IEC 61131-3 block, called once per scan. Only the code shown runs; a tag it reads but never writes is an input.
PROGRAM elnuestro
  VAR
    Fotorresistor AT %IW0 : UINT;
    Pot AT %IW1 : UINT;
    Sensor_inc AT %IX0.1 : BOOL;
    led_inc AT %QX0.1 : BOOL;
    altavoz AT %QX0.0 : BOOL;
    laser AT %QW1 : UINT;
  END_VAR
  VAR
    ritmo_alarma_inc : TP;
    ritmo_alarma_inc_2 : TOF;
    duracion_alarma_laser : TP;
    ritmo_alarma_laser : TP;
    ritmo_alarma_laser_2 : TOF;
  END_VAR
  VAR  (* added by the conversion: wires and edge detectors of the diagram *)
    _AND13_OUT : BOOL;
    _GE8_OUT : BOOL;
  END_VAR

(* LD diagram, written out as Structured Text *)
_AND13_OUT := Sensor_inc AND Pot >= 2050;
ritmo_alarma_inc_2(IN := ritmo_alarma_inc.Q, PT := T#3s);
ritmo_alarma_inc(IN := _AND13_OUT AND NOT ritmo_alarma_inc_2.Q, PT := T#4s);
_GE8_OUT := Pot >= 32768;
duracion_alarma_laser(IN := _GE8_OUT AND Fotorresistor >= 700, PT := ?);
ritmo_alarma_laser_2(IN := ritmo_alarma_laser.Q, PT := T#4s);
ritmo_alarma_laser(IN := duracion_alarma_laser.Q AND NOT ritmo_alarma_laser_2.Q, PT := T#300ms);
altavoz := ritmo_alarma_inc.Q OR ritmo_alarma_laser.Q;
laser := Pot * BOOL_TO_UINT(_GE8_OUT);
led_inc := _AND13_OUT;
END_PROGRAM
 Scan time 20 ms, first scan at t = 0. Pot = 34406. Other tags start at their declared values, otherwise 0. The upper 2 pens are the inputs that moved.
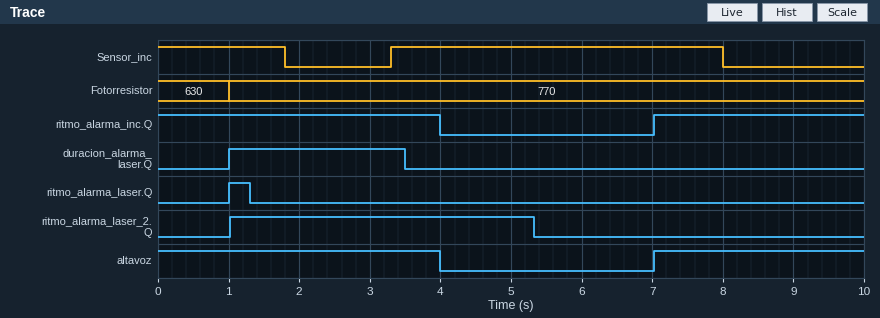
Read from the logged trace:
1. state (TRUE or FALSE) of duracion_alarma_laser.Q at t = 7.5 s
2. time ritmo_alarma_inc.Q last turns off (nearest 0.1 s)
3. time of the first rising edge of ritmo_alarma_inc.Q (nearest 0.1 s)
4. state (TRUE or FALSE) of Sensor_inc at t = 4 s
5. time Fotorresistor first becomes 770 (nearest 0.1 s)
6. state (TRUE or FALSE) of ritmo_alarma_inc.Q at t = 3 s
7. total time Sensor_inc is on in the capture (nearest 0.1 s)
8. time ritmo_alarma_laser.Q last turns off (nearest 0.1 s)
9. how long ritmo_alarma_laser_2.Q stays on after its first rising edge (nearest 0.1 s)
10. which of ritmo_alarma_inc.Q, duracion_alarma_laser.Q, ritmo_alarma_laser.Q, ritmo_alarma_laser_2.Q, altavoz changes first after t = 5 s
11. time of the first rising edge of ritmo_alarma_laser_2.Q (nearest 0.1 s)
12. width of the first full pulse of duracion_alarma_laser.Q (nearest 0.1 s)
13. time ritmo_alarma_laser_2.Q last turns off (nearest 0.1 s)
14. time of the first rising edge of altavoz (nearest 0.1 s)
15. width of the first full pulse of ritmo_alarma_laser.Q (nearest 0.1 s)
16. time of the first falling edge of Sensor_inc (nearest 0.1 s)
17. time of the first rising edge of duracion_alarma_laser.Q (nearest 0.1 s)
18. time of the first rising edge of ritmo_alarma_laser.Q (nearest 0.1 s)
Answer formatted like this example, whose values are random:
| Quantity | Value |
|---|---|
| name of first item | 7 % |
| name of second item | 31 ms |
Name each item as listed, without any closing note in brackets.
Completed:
| Quantity | Value |
|---|---|
| state (TRUE or FALSE) of duracion_alarma_laser.Q at t = 7.5 s | FALSE |
| time ritmo_alarma_inc.Q last turns off | 4.0 s |
| time of the first rising edge of ritmo_alarma_inc.Q | 7.0 s |
| state (TRUE or FALSE) of Sensor_inc at t = 4 s | TRUE |
| time Fotorresistor first becomes 770 | 1.0 s |
| state (TRUE or FALSE) of ritmo_alarma_inc.Q at t = 3 s | TRUE |
| total time Sensor_inc is on in the capture | 6.5 s |
| time ritmo_alarma_laser.Q last turns off | 1.3 s |
| how long ritmo_alarma_laser_2.Q stays on after its first rising edge | 4.3 s |
| which of ritmo_alarma_inc.Q, duracion_alarma_laser.Q, ritmo_alarma_laser.Q, ritmo_alarma_laser_2.Q, altavoz changes first after t = 5 s | ritmo_alarma_laser_2.Q |
| time of the first rising edge of ritmo_alarma_laser_2.Q | 1.0 s |
| width of the first full pulse of duracion_alarma_laser.Q | 2.5 s |
| time ritmo_alarma_laser_2.Q last turns off | 5.3 s |
| time of the first rising edge of altavoz | 7.0 s |
| width of the first full pulse of ritmo_alarma_laser.Q | 0.3 s |
| time of the first falling edge of Sensor_inc | 1.8 s |
| time of the first rising edge of duracion_alarma_laser.Q | 1.0 s |
| time of the first rising edge of ritmo_alarma_laser.Q | 1.0 s |
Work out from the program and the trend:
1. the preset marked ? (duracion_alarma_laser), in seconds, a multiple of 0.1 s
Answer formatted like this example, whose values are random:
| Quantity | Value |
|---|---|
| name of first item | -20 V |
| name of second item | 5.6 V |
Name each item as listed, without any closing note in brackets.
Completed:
| Quantity | Value |
|---|---|
| the preset marked ? (duracion_alarma_laser), in seconds, a multiple of 0.1 s | 2.5 s |
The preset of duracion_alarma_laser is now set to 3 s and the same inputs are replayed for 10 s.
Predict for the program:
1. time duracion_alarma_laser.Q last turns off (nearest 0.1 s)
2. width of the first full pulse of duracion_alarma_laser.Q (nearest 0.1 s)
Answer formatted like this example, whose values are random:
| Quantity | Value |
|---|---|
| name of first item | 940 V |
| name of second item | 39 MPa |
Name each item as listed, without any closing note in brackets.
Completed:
| Quantity | Value |
|---|---|
| time duracion_alarma_laser.Q last turns off | 4.0 s |
| width of the first full pulse of duracion_alarma_laser.Q | 3.0 s |
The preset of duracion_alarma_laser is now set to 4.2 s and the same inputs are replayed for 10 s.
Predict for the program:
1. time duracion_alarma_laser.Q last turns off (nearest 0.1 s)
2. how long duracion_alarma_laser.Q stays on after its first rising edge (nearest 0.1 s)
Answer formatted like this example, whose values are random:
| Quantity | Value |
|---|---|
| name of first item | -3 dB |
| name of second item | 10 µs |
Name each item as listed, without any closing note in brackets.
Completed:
| Quantity | Value |
|---|---|
| time duracion_alarma_laser.Q last turns off | 5.2 s |
| how long duracion_alarma_laser.Q stays on after its first rising edge | 4.2 s |
